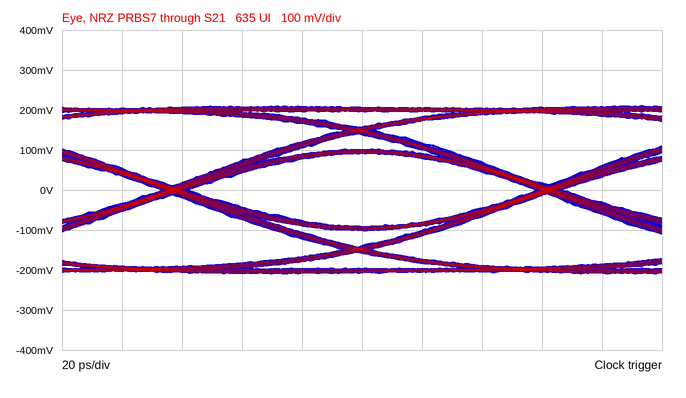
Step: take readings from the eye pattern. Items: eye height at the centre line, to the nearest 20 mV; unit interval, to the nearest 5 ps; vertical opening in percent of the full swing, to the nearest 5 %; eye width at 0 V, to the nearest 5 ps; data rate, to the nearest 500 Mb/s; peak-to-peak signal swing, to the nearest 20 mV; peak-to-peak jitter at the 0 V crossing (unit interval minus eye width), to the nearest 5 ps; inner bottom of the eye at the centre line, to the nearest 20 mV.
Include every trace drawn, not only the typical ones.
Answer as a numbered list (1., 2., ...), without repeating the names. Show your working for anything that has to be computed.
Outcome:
1. 180 mV
2. 125 ps
3. 180 mV / 420 mV ≈ 42.9 %, so 45 % to the nearest 5 %
4. 115 ps
5. 8.0 Gb/s
6. 420 mV
7. 10 ps
8. -100 mV
